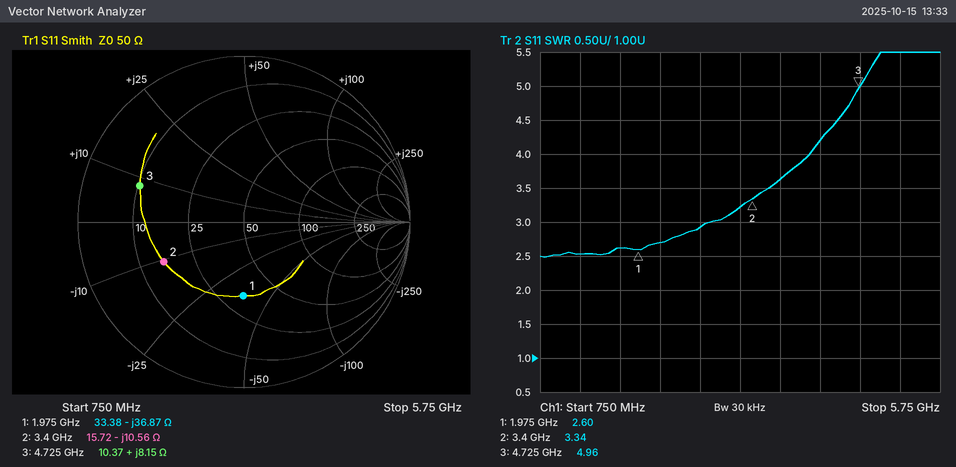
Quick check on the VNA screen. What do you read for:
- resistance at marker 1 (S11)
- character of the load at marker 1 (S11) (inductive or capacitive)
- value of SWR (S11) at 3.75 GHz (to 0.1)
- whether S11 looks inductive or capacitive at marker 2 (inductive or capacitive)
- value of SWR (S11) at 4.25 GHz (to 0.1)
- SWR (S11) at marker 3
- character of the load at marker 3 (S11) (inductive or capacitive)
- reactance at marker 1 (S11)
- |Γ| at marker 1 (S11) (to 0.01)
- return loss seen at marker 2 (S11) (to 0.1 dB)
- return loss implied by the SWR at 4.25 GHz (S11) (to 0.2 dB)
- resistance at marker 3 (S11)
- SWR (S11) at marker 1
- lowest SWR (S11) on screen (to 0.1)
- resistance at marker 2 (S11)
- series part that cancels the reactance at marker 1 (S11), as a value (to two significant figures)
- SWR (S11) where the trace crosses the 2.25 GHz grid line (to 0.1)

33.38 Ω
capacitive
3.6
capacitive
4.2
4.96
inductive
-36.87 Ω
0.44
5.4 dB
4.2 dB
10.37 Ω
2.60
2.5
15.72 Ω
3.0 nH
2.7
